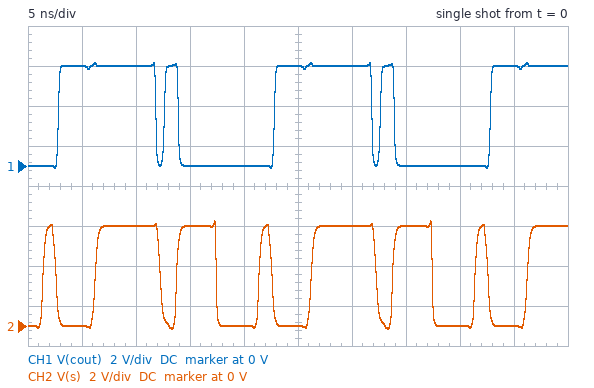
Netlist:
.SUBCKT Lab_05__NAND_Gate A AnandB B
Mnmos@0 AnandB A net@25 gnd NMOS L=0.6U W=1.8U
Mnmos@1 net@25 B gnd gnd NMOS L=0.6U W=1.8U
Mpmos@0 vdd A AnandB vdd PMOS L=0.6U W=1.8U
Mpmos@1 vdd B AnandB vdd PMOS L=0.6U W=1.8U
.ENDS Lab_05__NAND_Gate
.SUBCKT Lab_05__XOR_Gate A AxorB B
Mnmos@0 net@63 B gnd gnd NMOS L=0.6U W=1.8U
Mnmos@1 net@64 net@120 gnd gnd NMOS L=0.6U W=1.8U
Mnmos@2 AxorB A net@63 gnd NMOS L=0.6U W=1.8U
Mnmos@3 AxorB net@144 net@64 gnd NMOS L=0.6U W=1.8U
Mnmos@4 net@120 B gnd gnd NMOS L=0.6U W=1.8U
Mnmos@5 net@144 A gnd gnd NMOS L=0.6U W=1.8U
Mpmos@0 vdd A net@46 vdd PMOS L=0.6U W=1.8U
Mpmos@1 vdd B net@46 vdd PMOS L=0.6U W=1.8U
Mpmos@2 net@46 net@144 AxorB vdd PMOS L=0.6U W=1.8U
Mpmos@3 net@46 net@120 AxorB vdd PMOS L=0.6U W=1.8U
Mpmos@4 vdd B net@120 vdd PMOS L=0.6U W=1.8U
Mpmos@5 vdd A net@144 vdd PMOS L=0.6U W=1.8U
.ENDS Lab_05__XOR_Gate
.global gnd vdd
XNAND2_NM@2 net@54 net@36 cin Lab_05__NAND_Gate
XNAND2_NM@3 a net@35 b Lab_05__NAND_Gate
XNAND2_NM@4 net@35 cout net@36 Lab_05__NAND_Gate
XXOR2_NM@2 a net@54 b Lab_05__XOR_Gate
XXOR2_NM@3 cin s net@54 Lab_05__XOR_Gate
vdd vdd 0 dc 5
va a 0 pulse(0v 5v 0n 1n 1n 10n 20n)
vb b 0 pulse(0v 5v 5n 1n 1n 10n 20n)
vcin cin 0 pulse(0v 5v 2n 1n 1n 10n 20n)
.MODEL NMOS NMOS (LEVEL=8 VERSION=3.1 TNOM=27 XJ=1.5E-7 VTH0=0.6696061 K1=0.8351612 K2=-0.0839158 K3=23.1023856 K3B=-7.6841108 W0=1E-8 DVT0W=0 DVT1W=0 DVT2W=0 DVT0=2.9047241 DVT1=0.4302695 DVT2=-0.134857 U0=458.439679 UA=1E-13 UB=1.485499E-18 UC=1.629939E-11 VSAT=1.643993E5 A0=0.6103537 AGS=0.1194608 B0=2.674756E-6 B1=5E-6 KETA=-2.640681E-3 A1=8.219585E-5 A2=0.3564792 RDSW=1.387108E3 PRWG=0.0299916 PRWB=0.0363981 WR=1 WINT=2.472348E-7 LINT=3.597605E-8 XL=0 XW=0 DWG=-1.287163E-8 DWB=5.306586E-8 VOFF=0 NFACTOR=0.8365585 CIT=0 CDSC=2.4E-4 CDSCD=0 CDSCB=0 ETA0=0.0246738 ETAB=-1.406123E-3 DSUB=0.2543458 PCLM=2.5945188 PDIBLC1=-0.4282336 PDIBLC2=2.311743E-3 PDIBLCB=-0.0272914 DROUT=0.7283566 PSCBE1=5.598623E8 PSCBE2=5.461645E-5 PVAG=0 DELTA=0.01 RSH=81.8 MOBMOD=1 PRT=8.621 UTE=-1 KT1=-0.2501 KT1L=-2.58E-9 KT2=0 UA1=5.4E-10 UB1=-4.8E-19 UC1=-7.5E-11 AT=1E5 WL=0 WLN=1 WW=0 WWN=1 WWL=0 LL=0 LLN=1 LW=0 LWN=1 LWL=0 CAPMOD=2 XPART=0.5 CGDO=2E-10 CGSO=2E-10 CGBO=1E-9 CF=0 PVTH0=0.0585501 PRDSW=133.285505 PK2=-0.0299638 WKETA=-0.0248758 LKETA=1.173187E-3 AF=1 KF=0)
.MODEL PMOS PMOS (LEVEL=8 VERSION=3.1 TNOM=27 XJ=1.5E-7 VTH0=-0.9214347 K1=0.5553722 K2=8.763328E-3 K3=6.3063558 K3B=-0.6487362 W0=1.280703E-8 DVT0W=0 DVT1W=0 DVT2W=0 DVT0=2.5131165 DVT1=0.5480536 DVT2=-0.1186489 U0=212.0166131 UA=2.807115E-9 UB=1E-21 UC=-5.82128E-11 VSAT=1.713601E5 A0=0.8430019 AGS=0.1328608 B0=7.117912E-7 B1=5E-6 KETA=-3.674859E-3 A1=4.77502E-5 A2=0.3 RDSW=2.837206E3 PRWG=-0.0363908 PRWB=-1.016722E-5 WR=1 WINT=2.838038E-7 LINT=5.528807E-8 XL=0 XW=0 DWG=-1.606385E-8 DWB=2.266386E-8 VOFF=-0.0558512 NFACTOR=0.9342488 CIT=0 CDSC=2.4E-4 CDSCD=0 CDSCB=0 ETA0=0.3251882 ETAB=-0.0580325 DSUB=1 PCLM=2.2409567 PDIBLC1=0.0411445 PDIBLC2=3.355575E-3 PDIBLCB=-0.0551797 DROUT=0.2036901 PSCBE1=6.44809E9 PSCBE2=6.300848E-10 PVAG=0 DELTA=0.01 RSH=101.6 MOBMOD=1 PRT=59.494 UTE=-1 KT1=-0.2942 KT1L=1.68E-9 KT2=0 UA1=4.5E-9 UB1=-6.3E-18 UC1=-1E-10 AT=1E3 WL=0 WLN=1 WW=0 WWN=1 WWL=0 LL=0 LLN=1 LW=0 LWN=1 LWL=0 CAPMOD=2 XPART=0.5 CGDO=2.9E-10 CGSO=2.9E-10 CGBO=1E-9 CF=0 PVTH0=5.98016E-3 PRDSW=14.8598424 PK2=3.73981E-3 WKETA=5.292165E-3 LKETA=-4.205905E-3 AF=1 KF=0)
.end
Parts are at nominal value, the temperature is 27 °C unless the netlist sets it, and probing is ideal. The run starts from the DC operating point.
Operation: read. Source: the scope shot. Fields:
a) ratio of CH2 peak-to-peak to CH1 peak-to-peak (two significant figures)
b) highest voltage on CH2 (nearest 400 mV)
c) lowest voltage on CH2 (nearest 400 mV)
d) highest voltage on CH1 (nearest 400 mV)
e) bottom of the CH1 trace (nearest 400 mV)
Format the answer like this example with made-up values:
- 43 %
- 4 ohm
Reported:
- 1.0
- 5.2 V
- 0 V
- 5.2 V
- 0 V
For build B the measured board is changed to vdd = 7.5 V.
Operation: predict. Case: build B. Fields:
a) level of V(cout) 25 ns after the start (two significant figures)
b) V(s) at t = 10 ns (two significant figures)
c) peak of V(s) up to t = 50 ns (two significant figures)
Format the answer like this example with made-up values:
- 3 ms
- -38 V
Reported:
- 7.5 V
- 7.0 V
- 7.7 V
